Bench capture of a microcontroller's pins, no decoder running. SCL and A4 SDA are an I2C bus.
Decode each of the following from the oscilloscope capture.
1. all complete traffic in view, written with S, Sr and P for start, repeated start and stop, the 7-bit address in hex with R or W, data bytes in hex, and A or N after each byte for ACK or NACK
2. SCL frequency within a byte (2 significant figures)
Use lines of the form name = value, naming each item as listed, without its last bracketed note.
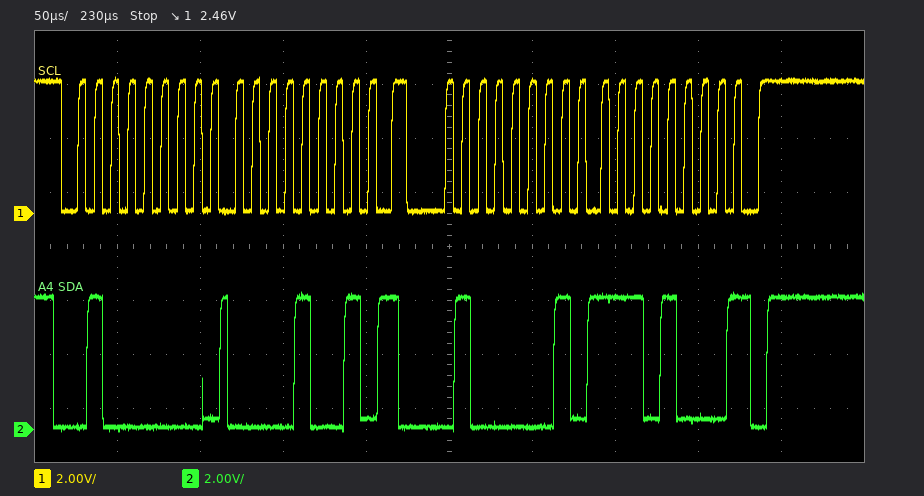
all complete traffic in view, written with S, Sr and P for start, repeated start and stop, the 7-bit address in hex with R or W, data bytes in hex, and A or N after each byte for ACK or NACK = S 20W A 09 A Sr 20R A E8 N P
SCL frequency within a byte = 100 kHz
